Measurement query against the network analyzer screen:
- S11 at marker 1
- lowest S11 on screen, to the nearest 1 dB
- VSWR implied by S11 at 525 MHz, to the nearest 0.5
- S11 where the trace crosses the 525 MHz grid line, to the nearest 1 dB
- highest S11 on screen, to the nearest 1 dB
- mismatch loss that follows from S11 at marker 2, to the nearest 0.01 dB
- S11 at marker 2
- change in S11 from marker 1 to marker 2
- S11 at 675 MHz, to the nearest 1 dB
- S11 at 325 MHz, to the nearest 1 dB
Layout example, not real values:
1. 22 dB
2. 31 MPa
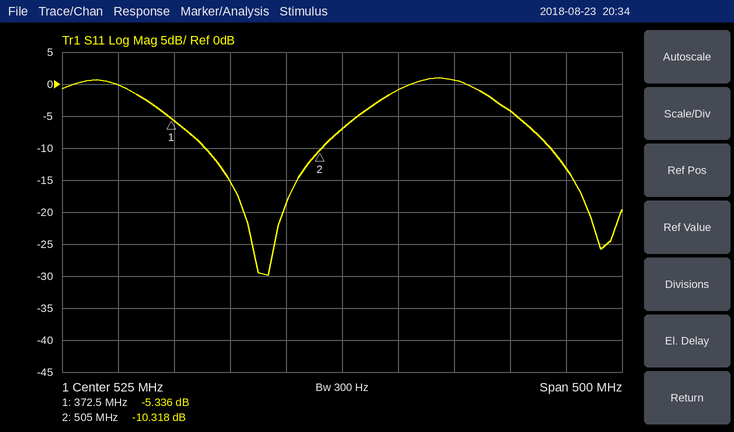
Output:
1. -5.336 dB
2. -30 dB
3. 2.5
4. -7 dB
5. 1 dB
6. 0.42 dB
7. -10.318 dB
8. -4.982 dB
9. -4 dB
10. 0 dB
